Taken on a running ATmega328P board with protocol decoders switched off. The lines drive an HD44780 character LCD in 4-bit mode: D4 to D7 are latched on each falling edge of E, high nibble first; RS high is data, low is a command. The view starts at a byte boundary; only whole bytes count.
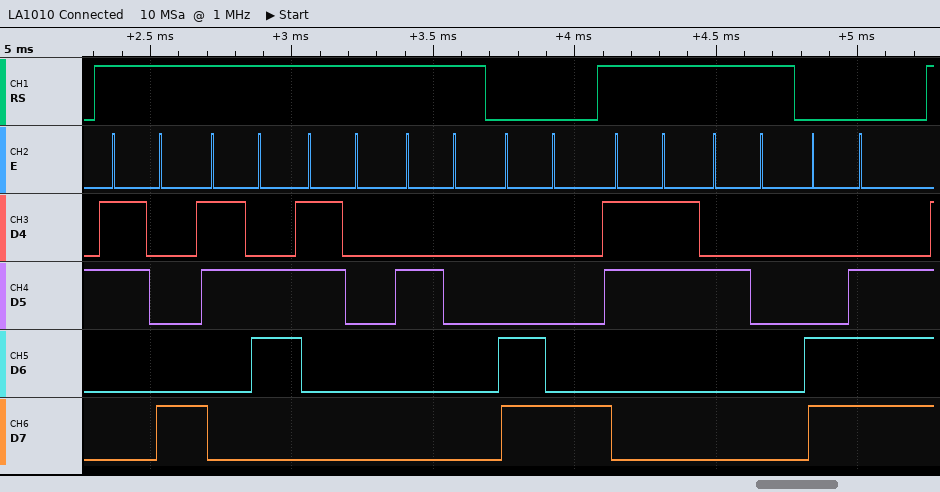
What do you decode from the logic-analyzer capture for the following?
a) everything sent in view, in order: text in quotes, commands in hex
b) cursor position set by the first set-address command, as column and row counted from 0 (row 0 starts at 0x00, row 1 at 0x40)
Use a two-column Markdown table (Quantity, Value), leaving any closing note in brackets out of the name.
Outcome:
| Quantity | Value |
|---|---|
| everything sent in view, in order: text in quotes, commands in hex | "860 " 0xC8 "3 " 0xCE |
| cursor position set by the first set-address command, as column and row counted from 0 | column 8, row 1 |
